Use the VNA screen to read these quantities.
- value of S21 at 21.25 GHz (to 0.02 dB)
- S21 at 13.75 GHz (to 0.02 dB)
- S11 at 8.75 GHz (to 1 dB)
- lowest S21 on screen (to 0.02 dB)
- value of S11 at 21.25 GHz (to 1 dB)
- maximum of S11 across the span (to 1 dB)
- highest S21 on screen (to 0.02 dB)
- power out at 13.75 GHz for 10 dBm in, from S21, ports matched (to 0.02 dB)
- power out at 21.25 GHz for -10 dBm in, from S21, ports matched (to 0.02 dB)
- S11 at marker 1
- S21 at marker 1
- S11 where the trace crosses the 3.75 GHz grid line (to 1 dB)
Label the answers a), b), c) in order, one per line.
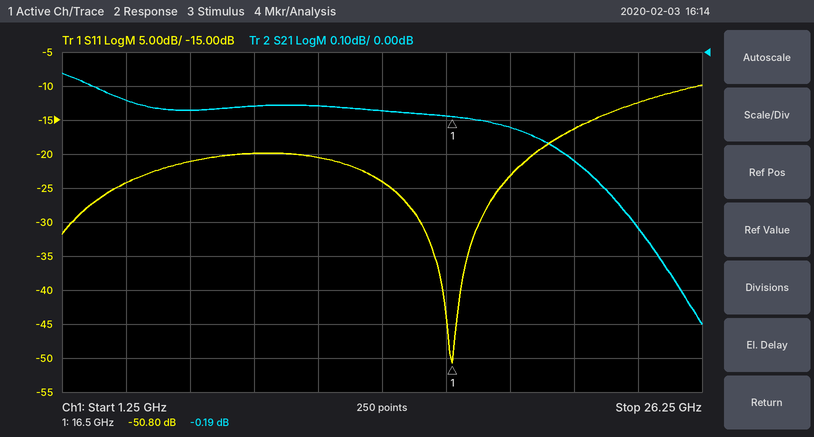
a) -0.32 dB
b) -0.18 dB
c) -20 dB
d) -0.80 dB
e) -16 dB
f) -10 dB
g) -0.06 dB
h) 9.82 dBm
i) -10.32 dBm
j) -50.80 dB
k) -0.19 dB
l) -24 dB
